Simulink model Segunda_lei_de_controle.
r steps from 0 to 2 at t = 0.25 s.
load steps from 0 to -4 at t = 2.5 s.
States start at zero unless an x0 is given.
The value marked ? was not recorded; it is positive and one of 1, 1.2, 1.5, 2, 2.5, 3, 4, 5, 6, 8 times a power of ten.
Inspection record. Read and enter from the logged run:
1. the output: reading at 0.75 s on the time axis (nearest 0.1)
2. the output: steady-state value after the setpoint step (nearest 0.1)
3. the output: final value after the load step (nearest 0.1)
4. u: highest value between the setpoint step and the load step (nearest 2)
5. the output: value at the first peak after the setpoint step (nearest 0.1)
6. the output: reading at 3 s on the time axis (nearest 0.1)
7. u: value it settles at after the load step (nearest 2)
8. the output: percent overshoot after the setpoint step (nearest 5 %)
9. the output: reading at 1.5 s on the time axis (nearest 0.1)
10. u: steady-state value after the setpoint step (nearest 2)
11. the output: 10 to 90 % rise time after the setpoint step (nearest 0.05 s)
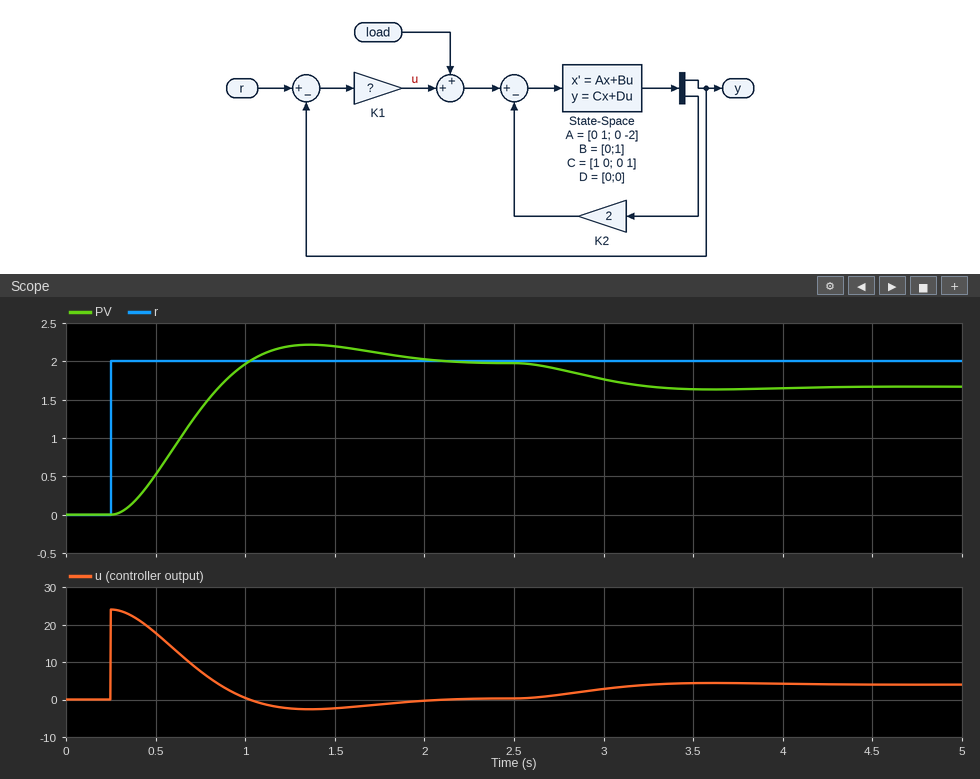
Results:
1.4
2.0
1.7
24
2.2
1.8
4
10 %
2.2
0
0.50 s
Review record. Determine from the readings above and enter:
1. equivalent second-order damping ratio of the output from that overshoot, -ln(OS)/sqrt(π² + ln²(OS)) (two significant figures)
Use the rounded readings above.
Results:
0.59
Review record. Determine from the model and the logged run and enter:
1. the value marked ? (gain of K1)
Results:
12
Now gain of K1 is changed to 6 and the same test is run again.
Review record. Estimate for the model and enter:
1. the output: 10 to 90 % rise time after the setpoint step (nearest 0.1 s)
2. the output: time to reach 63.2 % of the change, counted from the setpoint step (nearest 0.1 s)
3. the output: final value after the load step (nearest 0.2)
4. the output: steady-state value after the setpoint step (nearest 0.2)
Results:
1.0 s
0.8 s
1.4
2.0
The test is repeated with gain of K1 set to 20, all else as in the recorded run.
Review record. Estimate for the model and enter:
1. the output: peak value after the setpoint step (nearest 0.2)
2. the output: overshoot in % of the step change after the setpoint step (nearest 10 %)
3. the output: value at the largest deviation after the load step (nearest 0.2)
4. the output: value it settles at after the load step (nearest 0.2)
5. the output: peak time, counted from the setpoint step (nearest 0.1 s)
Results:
2.4
20 %
1.8
1.8
0.8 s
